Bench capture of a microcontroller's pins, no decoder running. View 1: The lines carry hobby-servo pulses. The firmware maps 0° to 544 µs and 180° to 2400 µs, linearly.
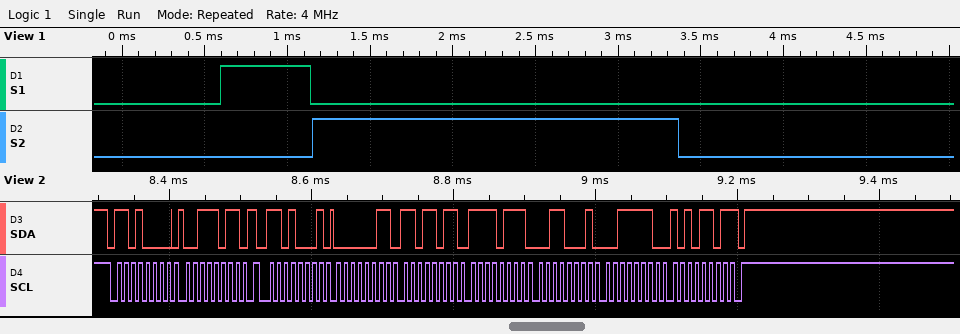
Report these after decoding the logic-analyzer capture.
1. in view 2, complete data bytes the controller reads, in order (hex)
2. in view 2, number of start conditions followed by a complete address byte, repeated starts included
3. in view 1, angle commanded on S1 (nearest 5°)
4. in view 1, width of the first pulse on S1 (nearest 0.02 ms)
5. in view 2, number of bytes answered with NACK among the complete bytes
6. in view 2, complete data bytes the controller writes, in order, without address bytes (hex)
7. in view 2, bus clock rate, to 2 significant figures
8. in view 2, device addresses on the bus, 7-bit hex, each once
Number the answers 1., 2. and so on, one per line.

1. 03 DB F7 31 3E AD
2. 2
3. 0°
4. 0.54 ms
5. 1
6. 3B
7. 100 kHz
8. 0x68
